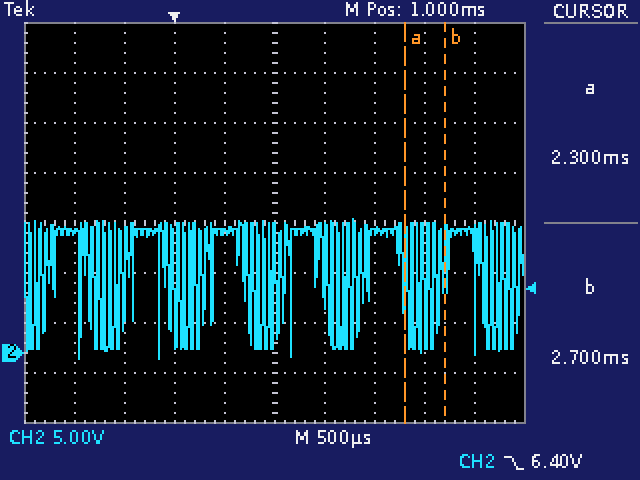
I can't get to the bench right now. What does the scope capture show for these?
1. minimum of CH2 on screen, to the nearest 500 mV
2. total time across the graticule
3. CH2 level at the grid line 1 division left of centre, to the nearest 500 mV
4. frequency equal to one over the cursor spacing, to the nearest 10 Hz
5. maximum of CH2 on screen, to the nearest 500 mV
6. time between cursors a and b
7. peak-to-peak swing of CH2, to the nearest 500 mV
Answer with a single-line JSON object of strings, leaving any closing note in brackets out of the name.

{"minimum of CH2 on screen, to the nearest 500 mV": "-500 mV", "total time across the graticule": "5 ms", "CH2 level at the grid line 1 division left of centre, to the nearest 500 mV": "12.0 V", "frequency equal to one over the cursor spacing, to the nearest 10 Hz": "2.50 kHz", "maximum of CH2 on screen, to the nearest 500 mV": "13.5 V", "time between cursors a and b": "400 µs", "peak-to-peak swing of CH2, to the nearest 500 mV": "14.0 V"}
